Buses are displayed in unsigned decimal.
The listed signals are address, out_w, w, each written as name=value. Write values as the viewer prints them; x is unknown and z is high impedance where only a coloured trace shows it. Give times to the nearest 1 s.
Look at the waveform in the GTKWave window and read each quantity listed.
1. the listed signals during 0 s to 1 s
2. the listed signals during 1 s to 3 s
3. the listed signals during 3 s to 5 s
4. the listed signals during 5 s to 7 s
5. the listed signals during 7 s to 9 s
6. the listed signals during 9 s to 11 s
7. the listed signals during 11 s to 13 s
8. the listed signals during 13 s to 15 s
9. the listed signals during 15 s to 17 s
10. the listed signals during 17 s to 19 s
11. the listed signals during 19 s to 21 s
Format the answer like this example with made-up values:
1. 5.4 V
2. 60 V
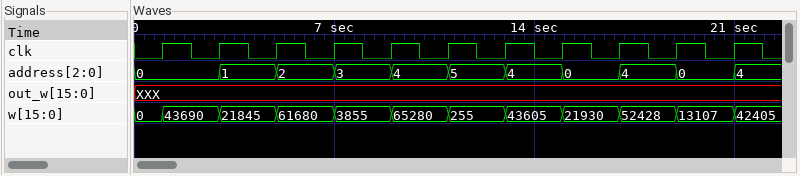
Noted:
1. address=0, out_w=XXX, w=0
2. address=0, out_w=XXX, w=43690
3. address=1, out_w=XXX, w=21845
4. address=2, out_w=XXX, w=61680
5. address=3, out_w=XXX, w=3855
6. address=4, out_w=XXX, w=65280
7. address=5, out_w=XXX, w=255
8. address=4, out_w=XXX, w=43605
9. address=0, out_w=XXX, w=21930
10. address=4, out_w=XXX, w=52428
11. address=0, out_w=XXX, w=13107
